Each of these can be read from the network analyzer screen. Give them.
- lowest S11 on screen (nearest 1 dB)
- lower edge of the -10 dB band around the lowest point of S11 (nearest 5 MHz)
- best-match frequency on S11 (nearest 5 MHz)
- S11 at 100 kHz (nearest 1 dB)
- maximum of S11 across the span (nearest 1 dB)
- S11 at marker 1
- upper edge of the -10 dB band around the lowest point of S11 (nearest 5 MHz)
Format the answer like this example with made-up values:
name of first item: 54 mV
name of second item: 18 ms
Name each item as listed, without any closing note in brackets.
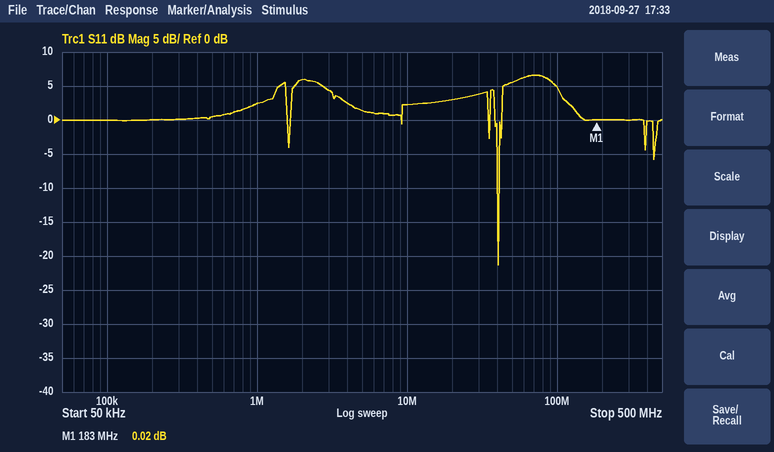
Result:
lowest S11 on screen: -21 dB
lower edge of the -10 dB band around the lowest point of S11: 40 MHz
best-match frequency on S11: 40 MHz
S11 at 100 kHz: 0 dB
maximum of S11 across the span: 7 dB
S11 at marker 1: 0.02 dB
upper edge of the -10 dB band around the lowest point of S11: 40 MHz
